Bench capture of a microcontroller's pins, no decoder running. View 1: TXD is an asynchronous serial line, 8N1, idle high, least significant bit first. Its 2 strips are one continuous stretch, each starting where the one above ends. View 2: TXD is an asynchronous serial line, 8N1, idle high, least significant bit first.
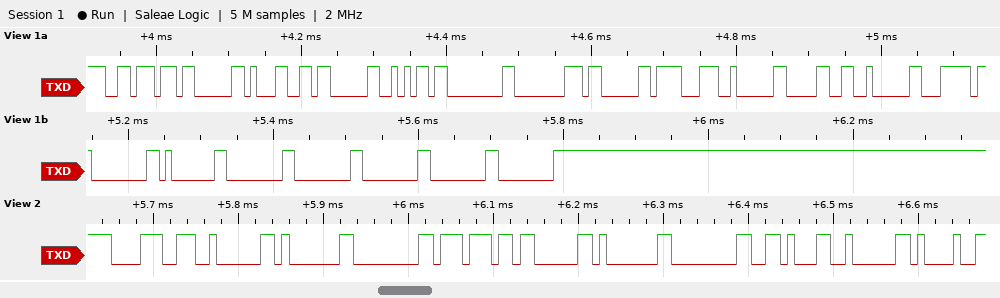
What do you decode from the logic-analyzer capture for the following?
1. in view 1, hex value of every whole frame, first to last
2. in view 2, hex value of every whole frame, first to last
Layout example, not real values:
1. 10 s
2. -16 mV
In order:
1. 76 03 31 03 6A 00 80 03 8F 02 30 02 7C 00 01 00 00 00 00 00
2. 38 02 01 00 77 03 01 00 16 02 21
